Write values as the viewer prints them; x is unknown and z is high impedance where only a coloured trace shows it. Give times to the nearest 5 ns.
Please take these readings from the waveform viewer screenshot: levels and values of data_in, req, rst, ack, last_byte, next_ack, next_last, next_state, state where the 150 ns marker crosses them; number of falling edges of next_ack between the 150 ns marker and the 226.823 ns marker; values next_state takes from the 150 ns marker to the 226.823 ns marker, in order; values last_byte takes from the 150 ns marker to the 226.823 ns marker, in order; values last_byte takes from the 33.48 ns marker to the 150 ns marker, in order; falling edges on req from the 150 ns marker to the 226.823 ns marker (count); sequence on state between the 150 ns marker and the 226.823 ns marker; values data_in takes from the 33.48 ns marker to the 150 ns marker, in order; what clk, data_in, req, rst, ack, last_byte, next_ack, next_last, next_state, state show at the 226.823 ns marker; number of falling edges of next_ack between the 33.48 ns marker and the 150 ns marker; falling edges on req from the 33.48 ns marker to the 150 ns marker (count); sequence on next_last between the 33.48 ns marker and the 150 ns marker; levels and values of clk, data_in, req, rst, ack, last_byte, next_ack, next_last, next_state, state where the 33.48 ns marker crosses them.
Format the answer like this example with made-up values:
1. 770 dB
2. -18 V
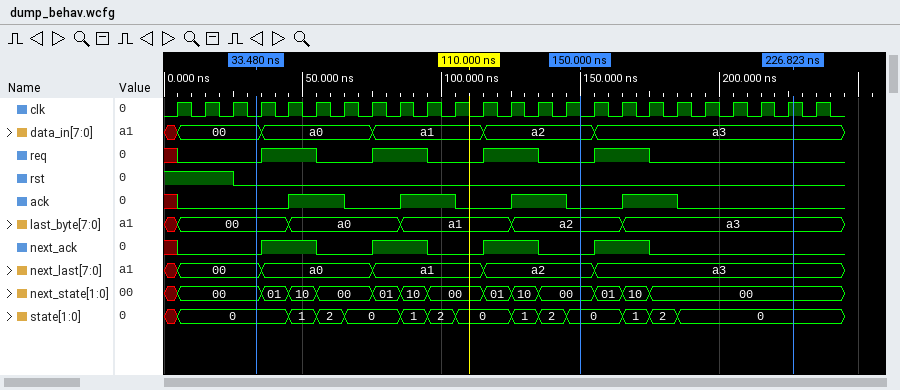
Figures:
1. data_in=a2, req=0, rst=0, ack=0, last_byte=a2, next_ack=0, next_last=a2, next_state=00, state=0
2. 1
3. 00, 01, 10, 00
4. a2, a3
5. 00, a0, a1, a2
6. 1
7. 0, 1, 2, 0
8. 00, a0, a1, a2
9. clk=1, data_in=a3, req=0, rst=0, ack=0, last_byte=a3, next_ack=0, next_last=a3, next_state=00, state=0
10. 3
11. 3
12. 00, a0, a1, a2
13. clk=0, data_in=00, req=0, rst=0, ack=0, last_byte=00, next_ack=0, next_last=00, next_state=00, state=0
